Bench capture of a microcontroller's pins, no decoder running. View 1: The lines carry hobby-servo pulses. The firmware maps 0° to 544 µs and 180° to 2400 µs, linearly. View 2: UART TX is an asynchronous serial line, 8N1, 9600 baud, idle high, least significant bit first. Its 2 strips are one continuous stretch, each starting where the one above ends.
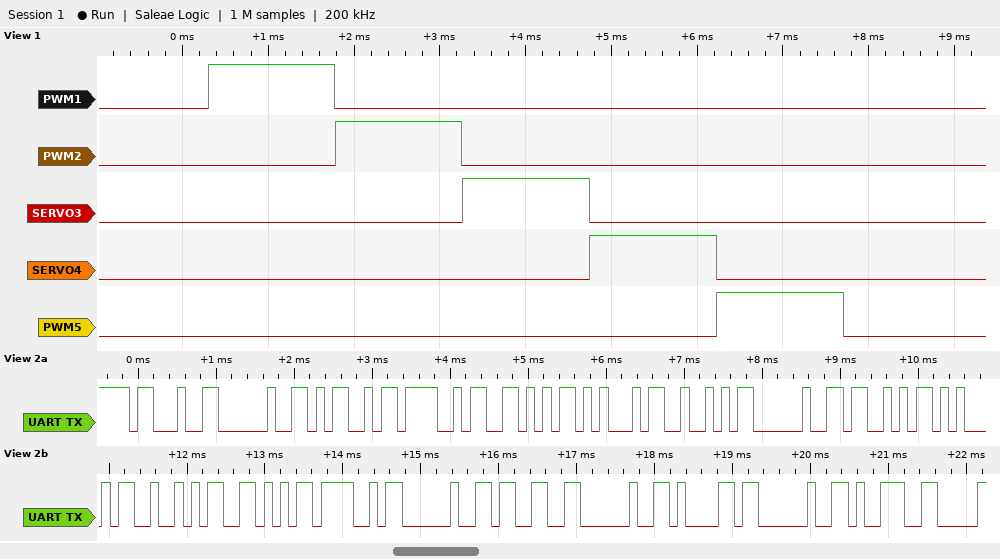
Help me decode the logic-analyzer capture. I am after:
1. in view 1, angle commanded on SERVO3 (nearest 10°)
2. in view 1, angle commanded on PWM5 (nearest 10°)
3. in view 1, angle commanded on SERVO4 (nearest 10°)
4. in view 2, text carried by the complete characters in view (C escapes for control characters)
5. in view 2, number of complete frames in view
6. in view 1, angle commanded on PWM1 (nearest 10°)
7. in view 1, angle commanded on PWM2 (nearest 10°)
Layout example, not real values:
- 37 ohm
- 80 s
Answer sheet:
- 90°
- 90°
- 90°
- "# MOVER SERVO 3 a 9"
- 19
- 90°
- 90°
